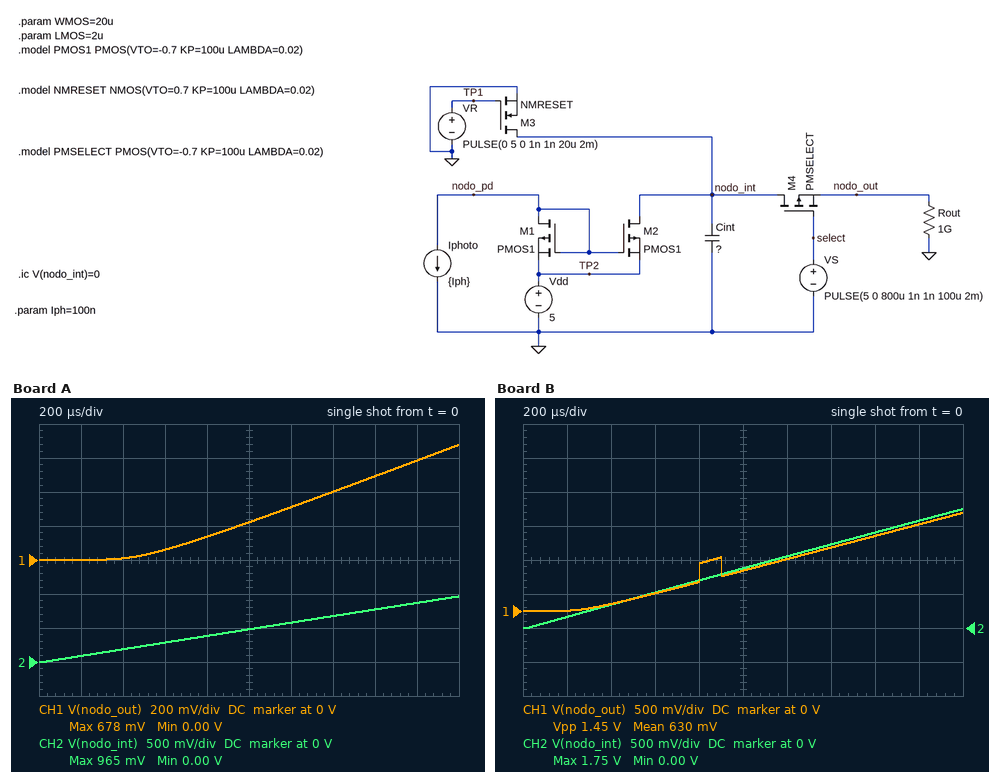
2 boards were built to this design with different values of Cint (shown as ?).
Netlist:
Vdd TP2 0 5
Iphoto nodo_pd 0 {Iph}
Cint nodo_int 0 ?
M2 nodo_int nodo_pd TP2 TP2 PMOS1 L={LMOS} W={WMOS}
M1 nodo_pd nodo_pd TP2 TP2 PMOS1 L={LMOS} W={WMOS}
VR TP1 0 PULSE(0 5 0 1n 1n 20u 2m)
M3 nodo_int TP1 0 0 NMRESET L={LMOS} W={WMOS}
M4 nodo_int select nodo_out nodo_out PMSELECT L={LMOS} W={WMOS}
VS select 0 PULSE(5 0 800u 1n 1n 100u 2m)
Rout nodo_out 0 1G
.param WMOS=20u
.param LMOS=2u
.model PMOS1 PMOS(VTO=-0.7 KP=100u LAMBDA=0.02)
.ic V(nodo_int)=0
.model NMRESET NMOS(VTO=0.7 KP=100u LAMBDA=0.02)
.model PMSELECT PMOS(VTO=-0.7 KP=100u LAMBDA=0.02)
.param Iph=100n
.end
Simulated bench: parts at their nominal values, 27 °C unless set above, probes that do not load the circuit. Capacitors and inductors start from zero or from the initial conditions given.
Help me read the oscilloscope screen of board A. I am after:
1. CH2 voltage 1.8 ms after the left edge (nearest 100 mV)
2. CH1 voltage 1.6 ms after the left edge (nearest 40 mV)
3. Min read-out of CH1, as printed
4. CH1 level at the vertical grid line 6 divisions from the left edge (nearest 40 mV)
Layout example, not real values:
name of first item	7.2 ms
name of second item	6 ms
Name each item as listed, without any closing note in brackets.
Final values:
CH2 voltage 1.8 ms after the left edge	900 mV
CH1 voltage 1.6 ms after the left edge	480 mV
Min read-out of CH1, as printed	0.00 V
CH1 level at the vertical grid line 6 divisions from the left edge	320 mV
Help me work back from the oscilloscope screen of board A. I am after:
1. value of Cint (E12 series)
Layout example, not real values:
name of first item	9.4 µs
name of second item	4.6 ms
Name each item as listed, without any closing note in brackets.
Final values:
value of Cint	220 pF
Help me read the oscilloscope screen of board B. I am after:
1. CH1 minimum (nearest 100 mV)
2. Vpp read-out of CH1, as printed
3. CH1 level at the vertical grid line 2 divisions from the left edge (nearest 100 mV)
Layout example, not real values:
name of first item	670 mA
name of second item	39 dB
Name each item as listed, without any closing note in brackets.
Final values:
CH1 minimum	0 V
Vpp read-out of CH1, as printed	1.45 V
CH1 level at the vertical grid line 2 divisions from the left edge	100 mV
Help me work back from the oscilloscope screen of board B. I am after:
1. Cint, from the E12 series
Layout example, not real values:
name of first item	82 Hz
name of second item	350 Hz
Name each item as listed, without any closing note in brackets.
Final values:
Cint, from the E12 series	120 pF
